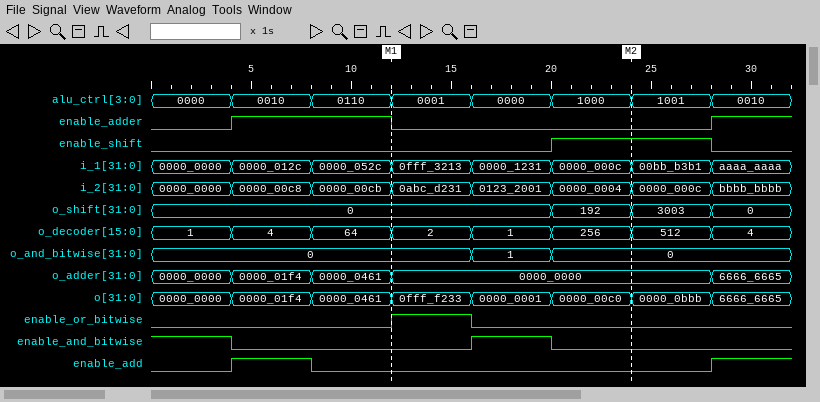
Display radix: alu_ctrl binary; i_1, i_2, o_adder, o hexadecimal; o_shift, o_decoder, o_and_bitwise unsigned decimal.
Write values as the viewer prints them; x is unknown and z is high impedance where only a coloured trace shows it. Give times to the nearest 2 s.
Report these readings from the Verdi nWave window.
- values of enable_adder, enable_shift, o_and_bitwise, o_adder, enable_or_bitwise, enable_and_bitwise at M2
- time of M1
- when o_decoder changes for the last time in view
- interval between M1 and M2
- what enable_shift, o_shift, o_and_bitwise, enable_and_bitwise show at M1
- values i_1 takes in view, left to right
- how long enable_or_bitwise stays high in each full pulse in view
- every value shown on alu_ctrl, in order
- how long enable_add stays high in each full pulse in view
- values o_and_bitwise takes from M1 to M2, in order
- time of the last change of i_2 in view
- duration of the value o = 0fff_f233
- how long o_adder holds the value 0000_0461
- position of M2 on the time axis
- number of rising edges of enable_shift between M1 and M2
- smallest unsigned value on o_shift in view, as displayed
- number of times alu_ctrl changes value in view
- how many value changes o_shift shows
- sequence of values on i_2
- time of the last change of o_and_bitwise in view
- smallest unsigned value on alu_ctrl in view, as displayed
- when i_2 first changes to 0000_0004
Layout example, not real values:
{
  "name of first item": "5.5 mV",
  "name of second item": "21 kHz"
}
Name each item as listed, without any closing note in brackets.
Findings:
{
  "values of enable_adder, enable_shift, o_and_bitwise, o_adder, enable_or_bitwise, enable_and_bitwise at M2": "enable_adder=0, enable_shift=1, o_and_bitwise=0, o_adder=0000_0000, enable_or_bitwise=0, enable_and_bitwise=0",
  "time of M1": "12 s",
  "when o_decoder changes for the last time in view": "28 s",
  "interval between M1 and M2": "12 s",
  "what enable_shift, o_shift, o_and_bitwise, enable_and_bitwise show at M1": "enable_shift=0, o_shift=0, o_and_bitwise=0, enable_and_bitwise=0",
  "values i_1 takes in view, left to right": "0000_0000, 0000_012c, 0000_052c, 0fff_3213, 0000_1231, 0000_000c, 00bb_b3b1, aaaa_aaaa",
  "how long enable_or_bitwise stays high in each full pulse in view": "4 s",
  "every value shown on alu_ctrl, in order": "0000, 0010, 0110, 0001, 0000, 1000, 1001, 0010",
  "how long enable_add stays high in each full pulse in view": "4 s",
  "values o_and_bitwise takes from M1 to M2, in order": "0, 1, 0",
  "time of the last change of i_2 in view": "28 s",
  "duration of the value o = 0fff_f233": "4 s",
  "how long o_adder holds the value 0000_0461": "4 s",
  "position of M2 on the time axis": "24 s",
  "number of rising edges of enable_shift between M1 and M2": "1",
  "smallest unsigned value on o_shift in view, as displayed": "0",
  "number of times alu_ctrl changes value in view": "7",
  "how many value changes o_shift shows": "3",
  "sequence of values on i_2": "0000_0000, 0000_00c8, 0000_00cb, 0abc_d231, 0123_2001, 0000_0004, 0000_000c, bbbb_bbbb",
  "time of the last change of o_and_bitwise in view": "20 s",
  "smallest unsigned value on alu_ctrl in view, as displayed": "0000",
  "when i_2 first changes to 0000_0004": "20 s"
}
